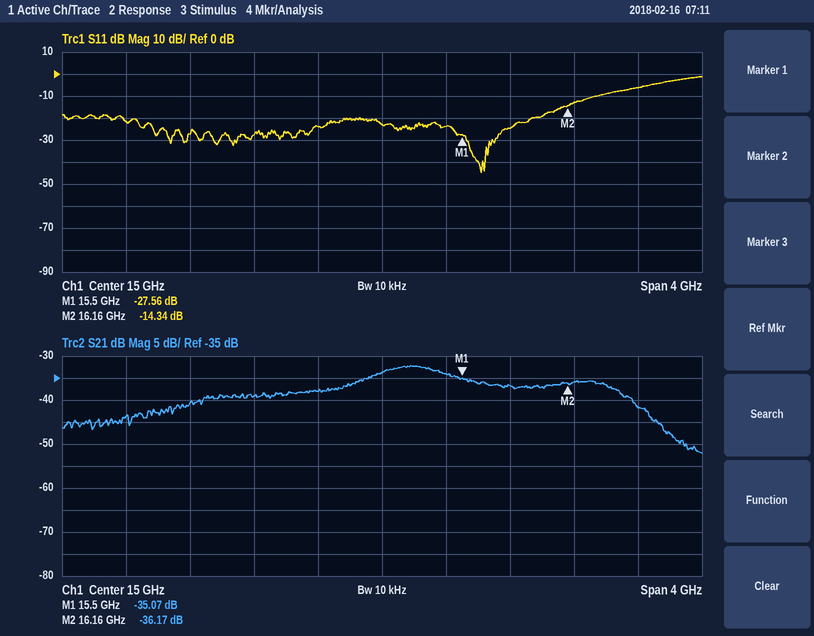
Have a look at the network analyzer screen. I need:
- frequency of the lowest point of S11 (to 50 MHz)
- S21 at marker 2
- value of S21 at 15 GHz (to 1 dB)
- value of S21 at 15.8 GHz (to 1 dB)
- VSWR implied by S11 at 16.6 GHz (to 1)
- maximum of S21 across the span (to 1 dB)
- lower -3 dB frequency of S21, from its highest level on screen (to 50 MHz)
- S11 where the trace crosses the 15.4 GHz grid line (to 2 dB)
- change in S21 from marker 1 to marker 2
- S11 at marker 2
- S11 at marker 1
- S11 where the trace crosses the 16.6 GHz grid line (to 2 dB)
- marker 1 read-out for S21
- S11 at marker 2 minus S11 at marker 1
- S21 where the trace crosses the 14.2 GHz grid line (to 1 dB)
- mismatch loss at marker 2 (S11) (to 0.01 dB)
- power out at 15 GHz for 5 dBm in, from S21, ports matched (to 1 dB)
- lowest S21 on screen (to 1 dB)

15.60 GHz
-36.17 dB
-34 dB
-37 dB
3
-32 dB
14.90 GHz
-24 dB
-1.10 dB
-14.34 dB
-27.56 dB
-6 dB
-35.07 dB
13.22 dB
-39 dB
0.16 dB
-29 dBm
-52 dB
